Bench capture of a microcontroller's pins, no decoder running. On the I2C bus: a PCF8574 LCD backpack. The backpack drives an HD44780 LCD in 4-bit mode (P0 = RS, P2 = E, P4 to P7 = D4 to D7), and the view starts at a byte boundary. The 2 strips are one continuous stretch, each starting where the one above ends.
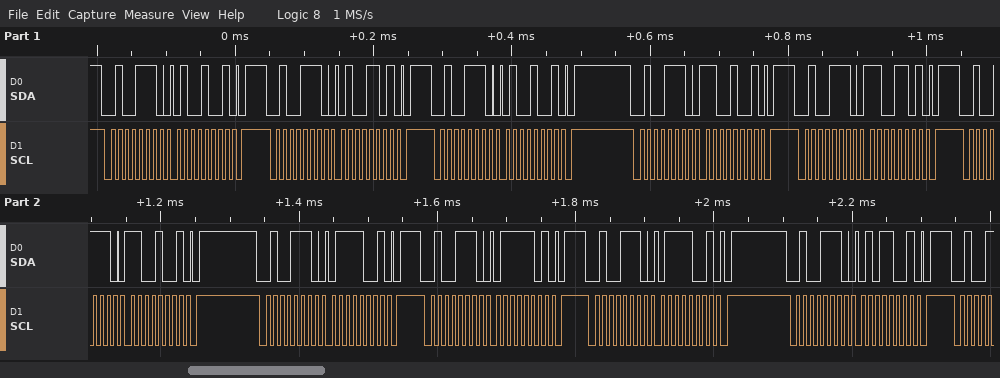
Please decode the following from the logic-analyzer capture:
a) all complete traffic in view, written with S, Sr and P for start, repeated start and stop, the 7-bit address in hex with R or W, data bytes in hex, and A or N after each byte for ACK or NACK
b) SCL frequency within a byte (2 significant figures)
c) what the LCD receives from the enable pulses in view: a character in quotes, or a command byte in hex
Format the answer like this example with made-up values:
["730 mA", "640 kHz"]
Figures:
["S 27W A 49 A P S 27W A 4D A P S 27W A 49 A P S 27W A C9 A P S 27W A CD A P S 27W A C9 A P S 27W A 79 A P S 27W A 7D A P S 27W A 79 A P S 27W A 59 A P", "100 kHz", "'L'"]
